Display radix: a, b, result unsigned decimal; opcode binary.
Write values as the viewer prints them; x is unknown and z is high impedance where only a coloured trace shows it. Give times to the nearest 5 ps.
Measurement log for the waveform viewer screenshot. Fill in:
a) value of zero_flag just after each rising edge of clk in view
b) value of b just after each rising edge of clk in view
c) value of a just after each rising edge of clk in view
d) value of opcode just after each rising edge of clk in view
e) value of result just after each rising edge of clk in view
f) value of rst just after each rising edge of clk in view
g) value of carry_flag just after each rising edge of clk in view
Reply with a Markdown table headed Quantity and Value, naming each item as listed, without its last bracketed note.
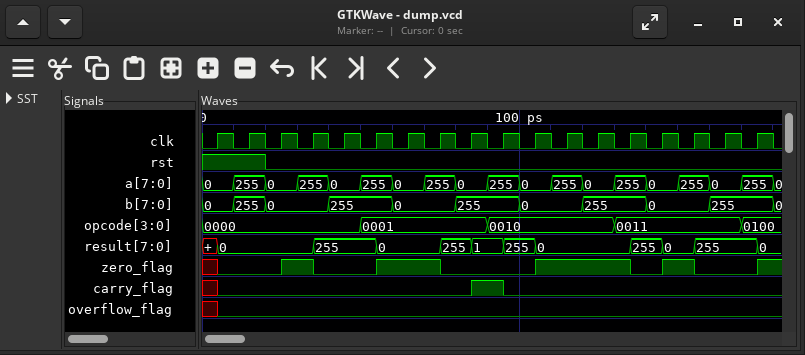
| Quantity | Value |
|---|---|
| value of zero_flag just after each rising edge of clk in view | 0 0 1 0 0 1 1 0 0 0 1 1 1 0 1 0 0 1 |
| value of b just after each rising edge of clk in view | 0, 255, 0, 0, 255, 255, 0, 0, 255, 255, 0, 0, 255, 255, 0, 0, 255, 255 |
| value of a just after each rising edge of clk in view | 0, 255, 0, 255, 0, 255, 0, 255, 0, 255, 0, 255, 0, 255, 0, 255, 0, 255 |
| value of opcode just after each rising edge of clk in view | 0000, 0000, 0000, 0000, 0000, 0001, 0001, 0001, 0001, 0010, 0010, 0010, 0010, 0011, 0011, 0011, 0011, 0100 |
| value of result just after each rising edge of clk in view | 0, 0, 0, 255, 255, 0, 0, 255, 1, 255, 0, 0, 0, 255, 0, 255, 255, 0 |
| value of rst just after each rising edge of clk in view | 1 1 0 0 0 0 0 0 0 0 0 0 0 0 0 0 0 0 |
| value of carry_flag just after each rising edge of clk in view | 0 0 0 0 0 0 0 0 1 0 0 0 0 0 0 0 0 0 |
